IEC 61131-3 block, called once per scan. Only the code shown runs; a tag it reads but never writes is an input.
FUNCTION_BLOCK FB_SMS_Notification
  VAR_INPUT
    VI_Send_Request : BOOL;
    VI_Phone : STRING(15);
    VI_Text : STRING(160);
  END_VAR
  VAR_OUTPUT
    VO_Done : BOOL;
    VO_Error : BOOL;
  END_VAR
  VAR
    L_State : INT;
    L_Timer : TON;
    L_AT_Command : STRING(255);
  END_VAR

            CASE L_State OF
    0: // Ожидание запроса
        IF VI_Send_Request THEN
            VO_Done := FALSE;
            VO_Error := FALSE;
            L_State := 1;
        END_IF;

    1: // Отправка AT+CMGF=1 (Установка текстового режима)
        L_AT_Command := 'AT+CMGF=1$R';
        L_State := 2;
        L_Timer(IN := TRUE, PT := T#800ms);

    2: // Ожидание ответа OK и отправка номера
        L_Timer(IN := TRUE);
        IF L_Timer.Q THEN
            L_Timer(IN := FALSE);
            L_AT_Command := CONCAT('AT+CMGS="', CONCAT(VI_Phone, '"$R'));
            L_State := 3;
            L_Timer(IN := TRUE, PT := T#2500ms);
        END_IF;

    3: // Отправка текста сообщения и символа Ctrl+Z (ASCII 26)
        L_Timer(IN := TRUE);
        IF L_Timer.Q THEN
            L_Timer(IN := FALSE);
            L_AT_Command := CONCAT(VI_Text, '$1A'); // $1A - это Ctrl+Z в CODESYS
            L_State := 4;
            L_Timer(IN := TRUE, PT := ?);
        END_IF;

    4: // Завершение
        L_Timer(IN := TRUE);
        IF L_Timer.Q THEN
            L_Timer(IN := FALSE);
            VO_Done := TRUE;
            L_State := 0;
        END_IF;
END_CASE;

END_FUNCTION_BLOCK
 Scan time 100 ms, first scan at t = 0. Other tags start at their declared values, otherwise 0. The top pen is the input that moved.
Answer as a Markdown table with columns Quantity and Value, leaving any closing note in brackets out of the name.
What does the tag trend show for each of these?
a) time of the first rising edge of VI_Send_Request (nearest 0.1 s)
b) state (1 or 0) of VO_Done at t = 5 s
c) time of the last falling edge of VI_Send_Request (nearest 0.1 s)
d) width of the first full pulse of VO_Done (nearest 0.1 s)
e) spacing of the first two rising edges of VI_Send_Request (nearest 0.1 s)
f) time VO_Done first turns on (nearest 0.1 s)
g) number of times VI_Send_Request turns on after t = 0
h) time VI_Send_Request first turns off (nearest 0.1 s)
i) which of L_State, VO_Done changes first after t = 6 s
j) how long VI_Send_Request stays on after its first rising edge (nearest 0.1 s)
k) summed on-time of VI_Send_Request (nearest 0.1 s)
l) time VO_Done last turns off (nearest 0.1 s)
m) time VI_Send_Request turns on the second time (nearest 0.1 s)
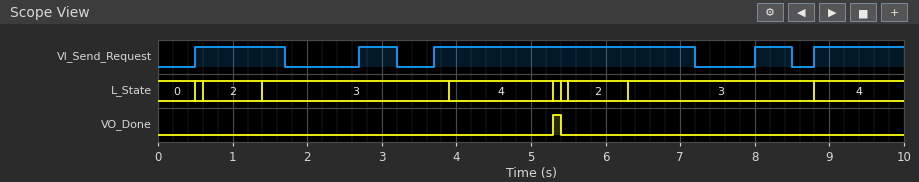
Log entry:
| Quantity | Value |
|---|---|
| time of the first rising edge of VI_Send_Request | 0.5 s |
| state (1 or 0) of VO_Done at t = 5 s | 0 |
| time of the last falling edge of VI_Send_Request | 8.5 s |
| width of the first full pulse of VO_Done | 0.1 s |
| spacing of the first two rising edges of VI_Send_Request | 2.2 s |
| time VO_Done first turns on | 5.3 s |
| number of times VI_Send_Request turns on after t = 0 | 5 |
| time VI_Send_Request first turns off | 1.7 s |
| which of L_State, VO_Done changes first after t = 6 s | L_State |
| how long VI_Send_Request stays on after its first rising edge | 1.2 s |
| summed on-time of VI_Send_Request | 6.9 s |
| time VO_Done last turns off | 5.4 s |
| time VI_Send_Request turns on the second time | 2.7 s |
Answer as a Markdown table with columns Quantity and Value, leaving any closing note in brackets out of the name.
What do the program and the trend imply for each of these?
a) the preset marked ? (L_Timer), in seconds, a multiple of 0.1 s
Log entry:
| Quantity | Value |
|---|---|
| the preset marked ? (L_Timer), in seconds, a multiple of 0.1 s | 1.4 s |
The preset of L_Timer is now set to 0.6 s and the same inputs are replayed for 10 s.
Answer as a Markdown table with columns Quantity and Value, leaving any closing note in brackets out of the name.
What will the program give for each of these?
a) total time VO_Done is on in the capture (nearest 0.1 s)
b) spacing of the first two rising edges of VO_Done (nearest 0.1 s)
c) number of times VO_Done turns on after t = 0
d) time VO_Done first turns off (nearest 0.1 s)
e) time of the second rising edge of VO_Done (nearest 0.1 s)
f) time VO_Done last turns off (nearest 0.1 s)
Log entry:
| Quantity | Value |
|---|---|
| total time VO_Done is on in the capture | 0.3 s |
| spacing of the first two rising edges of VO_Done | 4.1 s |
| number of times VO_Done turns on after t = 0 | 2 |
| time VO_Done first turns off | 4.6 s |
| time of the second rising edge of VO_Done | 8.6 s |
| time VO_Done last turns off | 8.8 s |
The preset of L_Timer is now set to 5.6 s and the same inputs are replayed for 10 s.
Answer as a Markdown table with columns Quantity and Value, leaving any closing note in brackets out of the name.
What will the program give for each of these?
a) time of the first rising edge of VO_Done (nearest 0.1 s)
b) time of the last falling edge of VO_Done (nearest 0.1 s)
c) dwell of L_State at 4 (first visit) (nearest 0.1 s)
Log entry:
| Quantity | Value |
|---|---|
| time of the first rising edge of VO_Done | 9.5 s |
| time of the last falling edge of VO_Done | 9.6 s |
| dwell of L_State at 4 (first visit) | 5.6 s |
